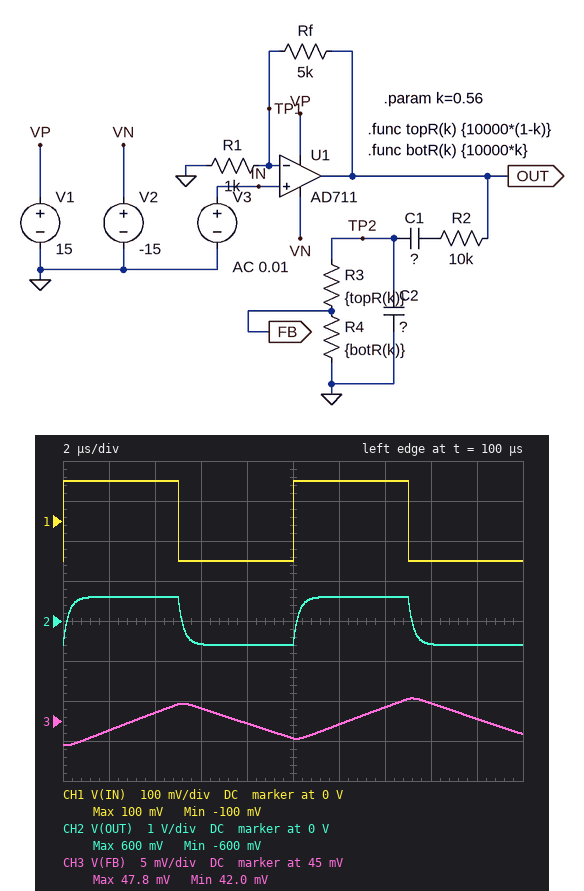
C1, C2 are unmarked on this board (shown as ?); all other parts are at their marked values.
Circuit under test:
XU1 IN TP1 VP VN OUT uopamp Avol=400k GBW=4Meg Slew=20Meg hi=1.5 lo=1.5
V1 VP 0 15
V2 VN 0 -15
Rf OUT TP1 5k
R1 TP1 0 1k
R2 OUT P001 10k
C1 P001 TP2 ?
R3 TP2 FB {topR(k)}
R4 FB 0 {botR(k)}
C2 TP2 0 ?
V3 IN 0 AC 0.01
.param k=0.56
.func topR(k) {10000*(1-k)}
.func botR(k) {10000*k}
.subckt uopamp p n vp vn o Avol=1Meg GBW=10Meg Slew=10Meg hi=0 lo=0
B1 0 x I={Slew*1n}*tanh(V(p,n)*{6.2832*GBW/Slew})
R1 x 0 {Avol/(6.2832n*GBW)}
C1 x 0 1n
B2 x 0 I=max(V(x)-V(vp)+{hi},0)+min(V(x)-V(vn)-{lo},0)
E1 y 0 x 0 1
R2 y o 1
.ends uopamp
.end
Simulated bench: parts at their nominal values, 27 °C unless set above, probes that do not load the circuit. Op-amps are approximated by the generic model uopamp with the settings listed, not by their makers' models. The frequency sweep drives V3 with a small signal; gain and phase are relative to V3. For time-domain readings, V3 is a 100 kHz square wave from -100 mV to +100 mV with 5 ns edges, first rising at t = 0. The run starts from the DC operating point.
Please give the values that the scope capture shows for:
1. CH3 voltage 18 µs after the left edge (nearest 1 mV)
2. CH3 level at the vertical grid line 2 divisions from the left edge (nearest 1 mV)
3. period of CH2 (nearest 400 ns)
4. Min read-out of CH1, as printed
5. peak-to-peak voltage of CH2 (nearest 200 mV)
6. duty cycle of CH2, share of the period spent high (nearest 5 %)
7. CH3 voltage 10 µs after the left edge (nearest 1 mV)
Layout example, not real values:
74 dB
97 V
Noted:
45 mV
46 mV
10.0 µs
-100 mV
1.2 V
50 %
43 mV
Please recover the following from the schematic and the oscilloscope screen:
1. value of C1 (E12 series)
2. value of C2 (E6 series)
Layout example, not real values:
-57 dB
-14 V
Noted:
8.2 nF
33 nF
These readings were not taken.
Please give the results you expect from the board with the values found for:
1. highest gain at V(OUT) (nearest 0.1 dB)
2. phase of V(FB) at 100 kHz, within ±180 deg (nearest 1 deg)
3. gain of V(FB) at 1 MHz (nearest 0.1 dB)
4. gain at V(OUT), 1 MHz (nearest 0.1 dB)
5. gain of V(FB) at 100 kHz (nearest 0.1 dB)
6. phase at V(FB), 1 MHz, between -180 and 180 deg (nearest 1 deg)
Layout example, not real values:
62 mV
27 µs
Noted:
15.6 dB
-97 deg
-60.9 dB
10.4 dB
-35.9 dB
-146 deg
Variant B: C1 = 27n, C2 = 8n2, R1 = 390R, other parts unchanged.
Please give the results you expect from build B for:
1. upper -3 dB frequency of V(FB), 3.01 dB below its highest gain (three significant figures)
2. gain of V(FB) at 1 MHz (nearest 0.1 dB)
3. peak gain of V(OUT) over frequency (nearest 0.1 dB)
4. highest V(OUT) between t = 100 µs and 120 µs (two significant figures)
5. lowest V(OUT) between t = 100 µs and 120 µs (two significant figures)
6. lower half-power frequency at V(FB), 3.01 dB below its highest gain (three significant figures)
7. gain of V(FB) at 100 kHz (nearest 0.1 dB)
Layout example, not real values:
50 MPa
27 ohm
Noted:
4.71 kHz
-47.6 dB
22.8 dB
1.4 V
-1.4 V
243 Hz
-17.0 dB
